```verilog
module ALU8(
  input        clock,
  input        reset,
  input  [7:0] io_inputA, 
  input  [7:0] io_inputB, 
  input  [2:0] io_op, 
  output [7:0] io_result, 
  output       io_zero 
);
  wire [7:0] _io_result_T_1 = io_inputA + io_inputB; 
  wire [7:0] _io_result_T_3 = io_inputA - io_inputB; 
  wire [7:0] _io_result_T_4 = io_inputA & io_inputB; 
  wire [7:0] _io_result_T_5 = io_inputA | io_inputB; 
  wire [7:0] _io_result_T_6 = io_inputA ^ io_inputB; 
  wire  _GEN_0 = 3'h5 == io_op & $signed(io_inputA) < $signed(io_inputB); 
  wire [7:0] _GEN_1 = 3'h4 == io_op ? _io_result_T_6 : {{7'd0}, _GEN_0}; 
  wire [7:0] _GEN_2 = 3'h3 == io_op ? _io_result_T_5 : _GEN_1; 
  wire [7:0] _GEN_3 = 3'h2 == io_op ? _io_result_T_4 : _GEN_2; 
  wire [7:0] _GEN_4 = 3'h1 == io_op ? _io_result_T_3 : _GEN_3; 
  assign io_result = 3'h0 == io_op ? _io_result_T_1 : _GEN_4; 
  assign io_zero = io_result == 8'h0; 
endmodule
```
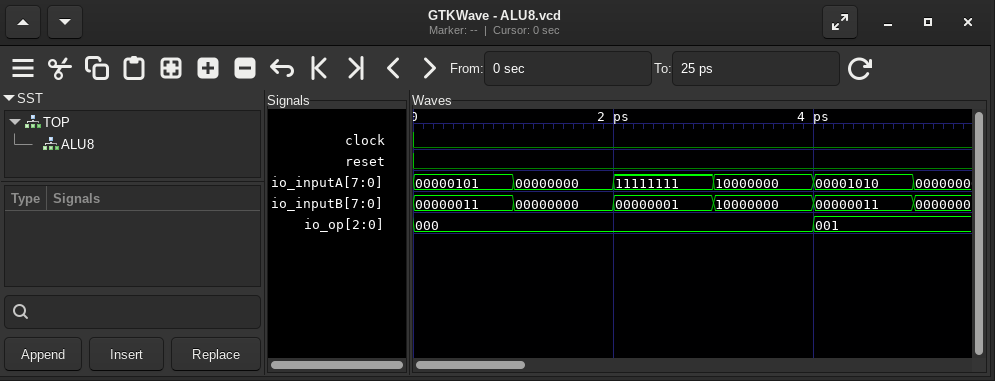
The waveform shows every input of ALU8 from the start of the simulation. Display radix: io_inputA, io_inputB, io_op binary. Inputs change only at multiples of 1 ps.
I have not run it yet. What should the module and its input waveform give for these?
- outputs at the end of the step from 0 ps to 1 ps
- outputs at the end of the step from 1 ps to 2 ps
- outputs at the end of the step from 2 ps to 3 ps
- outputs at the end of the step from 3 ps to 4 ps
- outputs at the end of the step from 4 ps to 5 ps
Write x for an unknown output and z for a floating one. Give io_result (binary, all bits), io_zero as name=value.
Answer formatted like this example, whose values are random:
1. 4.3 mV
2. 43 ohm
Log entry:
1. io_result=00001000, io_zero=0
2. io_result=00000000, io_zero=1
3. io_result=00000000, io_zero=1
4. io_result=00000000, io_zero=1
5. io_result=00000111, io_zero=0
